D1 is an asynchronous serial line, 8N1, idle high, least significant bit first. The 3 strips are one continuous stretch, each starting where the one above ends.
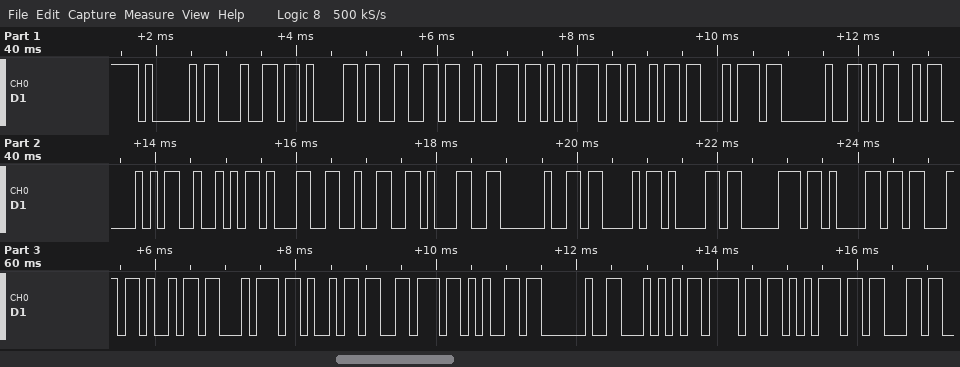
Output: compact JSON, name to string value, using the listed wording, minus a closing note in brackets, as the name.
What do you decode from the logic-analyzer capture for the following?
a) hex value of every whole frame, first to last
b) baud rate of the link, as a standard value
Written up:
{"hex value of every whole frame, first to last": "0x41 0x64 0x61 0x66 0x72 0x75 0x69 0x74 0x20 0x4D 0x50 0x52 0x31 0x32 0x31 0x20 0x43 0x61 0x70 0x61 0x63 0x69 0x74 0x69 0x76 0x65 0x20 0x54 0x6F 0x75 0x63", "baud rate of the link, as a standard value": "9600 baud"}
